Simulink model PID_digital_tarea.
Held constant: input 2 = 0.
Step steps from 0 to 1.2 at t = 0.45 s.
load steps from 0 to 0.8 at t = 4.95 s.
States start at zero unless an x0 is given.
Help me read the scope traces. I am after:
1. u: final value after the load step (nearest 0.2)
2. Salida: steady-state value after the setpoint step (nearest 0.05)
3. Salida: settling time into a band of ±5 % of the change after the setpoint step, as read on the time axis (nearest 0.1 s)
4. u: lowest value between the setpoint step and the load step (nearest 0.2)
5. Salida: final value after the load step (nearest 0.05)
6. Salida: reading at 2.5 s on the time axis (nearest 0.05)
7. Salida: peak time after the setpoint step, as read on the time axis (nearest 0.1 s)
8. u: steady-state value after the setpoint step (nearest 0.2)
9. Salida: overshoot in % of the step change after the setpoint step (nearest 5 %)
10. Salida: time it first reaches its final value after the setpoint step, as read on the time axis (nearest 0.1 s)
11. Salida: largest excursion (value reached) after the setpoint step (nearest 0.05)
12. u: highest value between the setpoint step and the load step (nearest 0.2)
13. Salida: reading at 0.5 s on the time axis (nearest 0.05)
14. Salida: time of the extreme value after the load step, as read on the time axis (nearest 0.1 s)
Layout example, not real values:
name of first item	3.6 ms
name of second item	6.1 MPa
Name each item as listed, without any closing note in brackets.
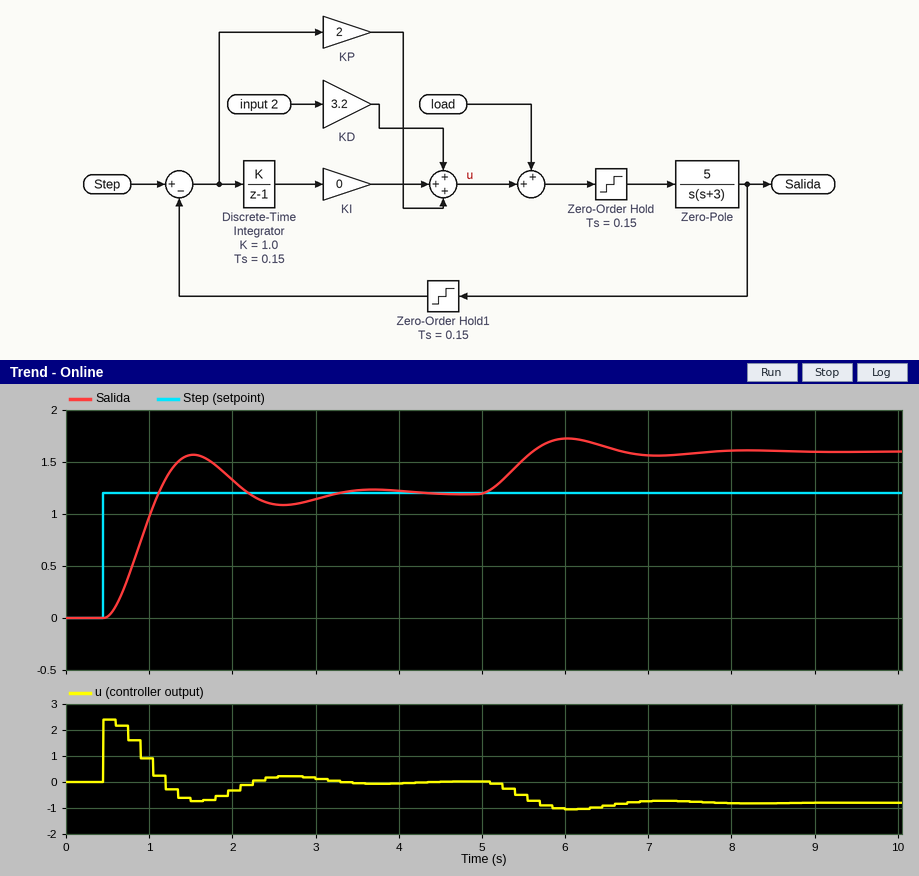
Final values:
u: final value after the load step	-0.8
Salida: steady-state value after the setpoint step	1.20
Salida: settling time into a band of ±5 % of the change after the setpoint step, as read on the time axis	3.0 s
u: lowest value between the setpoint step and the load step	-0.8
Salida: final value after the load step	1.60
Salida: reading at 2.5 s on the time axis	1.10
Salida: peak time after the setpoint step, as read on the time axis	1.5 s
u: steady-state value after the setpoint step	0.0
Salida: overshoot in % of the step change after the setpoint step	30 %
Salida: time it first reaches its final value after the setpoint step, as read on the time axis	1.1 s
Salida: largest excursion (value reached) after the setpoint step	1.55
u: highest value between the setpoint step and the load step	2.4
Salida: reading at 0.5 s on the time axis	0.00
Salida: time of the extreme value after the load step, as read on the time axis	6.0 s
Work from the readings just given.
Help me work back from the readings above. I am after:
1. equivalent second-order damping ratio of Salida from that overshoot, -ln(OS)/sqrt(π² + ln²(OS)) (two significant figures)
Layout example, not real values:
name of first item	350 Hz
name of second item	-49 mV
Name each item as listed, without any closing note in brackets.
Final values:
equivalent second-order damping ratio of Salida from that overshoot, -ln(OS)/sqrt(π² + ln²(OS))	0.36
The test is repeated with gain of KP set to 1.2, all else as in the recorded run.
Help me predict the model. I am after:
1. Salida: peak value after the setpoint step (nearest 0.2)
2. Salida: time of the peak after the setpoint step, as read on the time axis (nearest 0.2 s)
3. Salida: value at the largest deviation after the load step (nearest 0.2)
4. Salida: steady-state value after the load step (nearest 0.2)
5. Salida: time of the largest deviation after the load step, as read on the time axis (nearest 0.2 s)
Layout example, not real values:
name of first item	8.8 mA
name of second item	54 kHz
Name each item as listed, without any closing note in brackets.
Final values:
Salida: peak value after the setpoint step	1.4
Salida: time of the peak after the setpoint step, as read on the time axis	2.0 s
Salida: value at the largest deviation after the load step	2.0
Salida: steady-state value after the load step	1.8
Salida: time of the largest deviation after the load step, as read on the time axis	6.4 s
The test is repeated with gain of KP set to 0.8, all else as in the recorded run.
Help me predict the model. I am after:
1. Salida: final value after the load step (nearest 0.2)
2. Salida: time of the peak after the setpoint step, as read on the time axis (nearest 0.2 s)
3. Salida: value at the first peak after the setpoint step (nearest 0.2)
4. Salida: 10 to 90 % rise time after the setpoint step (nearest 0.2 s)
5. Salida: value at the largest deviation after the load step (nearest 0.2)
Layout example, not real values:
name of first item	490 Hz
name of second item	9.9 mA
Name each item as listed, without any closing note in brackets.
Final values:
Salida: final value after the load step	2.2
Salida: time of the peak after the setpoint step, as read on the time axis	2.6 s
Salida: value at the first peak after the setpoint step	1.2
Salida: 10 to 90 % rise time after the setpoint step	1.0 s
Salida: value at the largest deviation after the load step	2.2
